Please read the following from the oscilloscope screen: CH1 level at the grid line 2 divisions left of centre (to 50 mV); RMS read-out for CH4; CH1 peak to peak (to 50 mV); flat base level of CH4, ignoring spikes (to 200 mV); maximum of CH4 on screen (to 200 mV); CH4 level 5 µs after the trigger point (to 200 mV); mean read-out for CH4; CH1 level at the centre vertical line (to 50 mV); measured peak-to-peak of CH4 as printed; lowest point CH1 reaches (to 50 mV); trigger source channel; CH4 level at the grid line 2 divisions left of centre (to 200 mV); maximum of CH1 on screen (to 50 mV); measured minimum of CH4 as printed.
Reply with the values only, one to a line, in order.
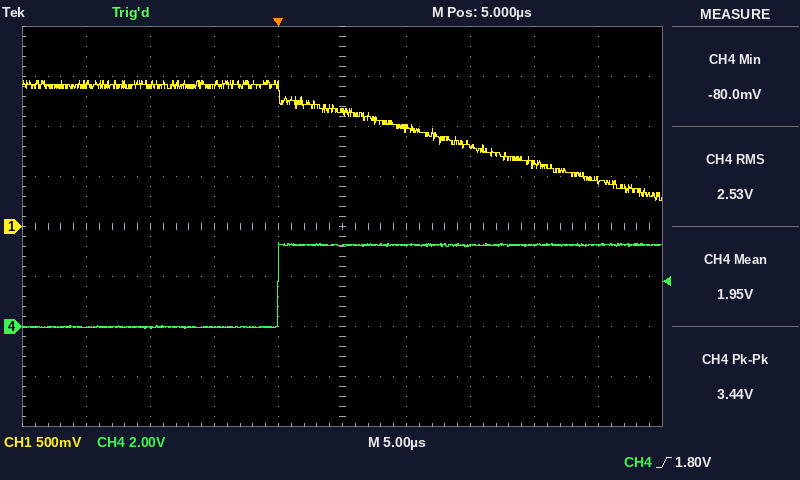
1.40 V
2.53 V
1.20 V
0.0 V
3.4 V
3.2 V
1.95 V
1.15 V
3.44 V
250 mV
CH4
0.0 V
1.45 V
-80.0 mV
